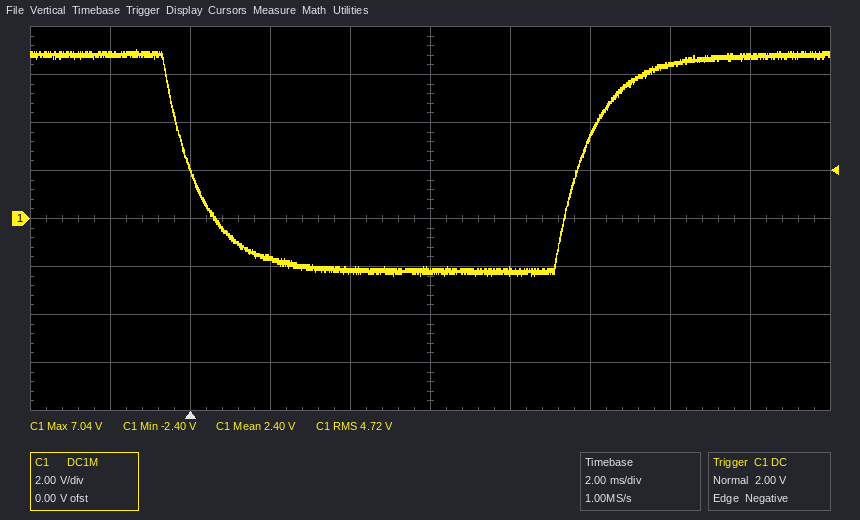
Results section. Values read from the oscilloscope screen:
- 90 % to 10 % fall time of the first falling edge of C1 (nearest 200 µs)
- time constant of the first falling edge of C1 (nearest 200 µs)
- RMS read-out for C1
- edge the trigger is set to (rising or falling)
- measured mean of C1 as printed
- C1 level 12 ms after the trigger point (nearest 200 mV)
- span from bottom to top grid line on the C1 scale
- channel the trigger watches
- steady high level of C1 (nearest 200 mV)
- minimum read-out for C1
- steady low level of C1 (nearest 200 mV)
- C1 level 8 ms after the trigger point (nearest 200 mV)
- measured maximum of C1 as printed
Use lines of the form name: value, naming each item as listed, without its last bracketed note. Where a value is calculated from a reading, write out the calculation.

90 % to 10 % fall time of the first falling edge of C1: 2.0 ms
time constant of the first falling edge of C1: 2.0 ms / 2.2 ≈ 0.909 ms, so 1.0 ms to the nearest 200 µs
RMS read-out for C1: 4.72 V
edge the trigger is set to: falling
measured mean of C1 as printed: 2.40 V
C1 level 12 ms after the trigger point: 6.4 V
span from bottom to top grid line on the C1 scale: 16 V
channel the trigger watches: C1
steady high level of C1: 6.8 V
minimum read-out for C1: -2.40 V
steady low level of C1: -2.2 V
C1 level 8 ms after the trigger point: -2.2 V
measured maximum of C1 as printed: 7.04 V
